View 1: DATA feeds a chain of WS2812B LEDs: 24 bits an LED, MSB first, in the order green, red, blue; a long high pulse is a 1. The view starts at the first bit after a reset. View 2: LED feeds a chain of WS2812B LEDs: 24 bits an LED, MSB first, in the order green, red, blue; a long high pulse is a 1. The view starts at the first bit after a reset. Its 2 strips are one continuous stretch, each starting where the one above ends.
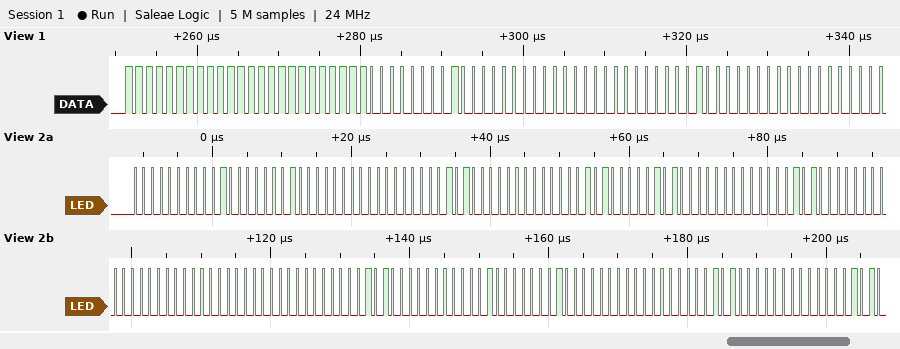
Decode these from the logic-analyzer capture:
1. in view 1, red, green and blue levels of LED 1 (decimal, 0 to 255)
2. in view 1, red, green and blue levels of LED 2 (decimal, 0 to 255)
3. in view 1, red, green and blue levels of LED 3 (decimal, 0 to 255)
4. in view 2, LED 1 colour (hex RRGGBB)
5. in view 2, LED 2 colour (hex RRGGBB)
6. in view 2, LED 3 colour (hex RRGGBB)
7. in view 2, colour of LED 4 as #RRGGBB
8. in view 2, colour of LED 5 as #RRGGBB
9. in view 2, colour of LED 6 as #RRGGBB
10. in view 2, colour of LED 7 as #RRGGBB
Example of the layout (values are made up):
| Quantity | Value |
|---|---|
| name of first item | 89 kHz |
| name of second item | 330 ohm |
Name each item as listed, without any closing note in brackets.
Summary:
| Quantity | Value |
|---|---|
| in view 1, red, green and blue levels of LED 1 | 255, 255, 255 |
| in view 1, red, green and blue levels of LED 2 | 128, 0, 0 |
| in view 1, red, green and blue levels of LED 3 | 128, 0, 0 |
| in view 2, LED 1 colour | #200020 |
| in view 2, LED 2 colour | #0A0000 |
| in view 2, LED 3 colour | #0A0A00 |
| in view 2, colour of LED 4 as #RRGGBB | #000A00 |
| in view 2, colour of LED 5 as #RRGGBB | #00000A |
| in view 2, colour of LED 6 as #RRGGBB | #200020 |
| in view 2, colour of LED 7 as #RRGGBB | #0A0000 |
